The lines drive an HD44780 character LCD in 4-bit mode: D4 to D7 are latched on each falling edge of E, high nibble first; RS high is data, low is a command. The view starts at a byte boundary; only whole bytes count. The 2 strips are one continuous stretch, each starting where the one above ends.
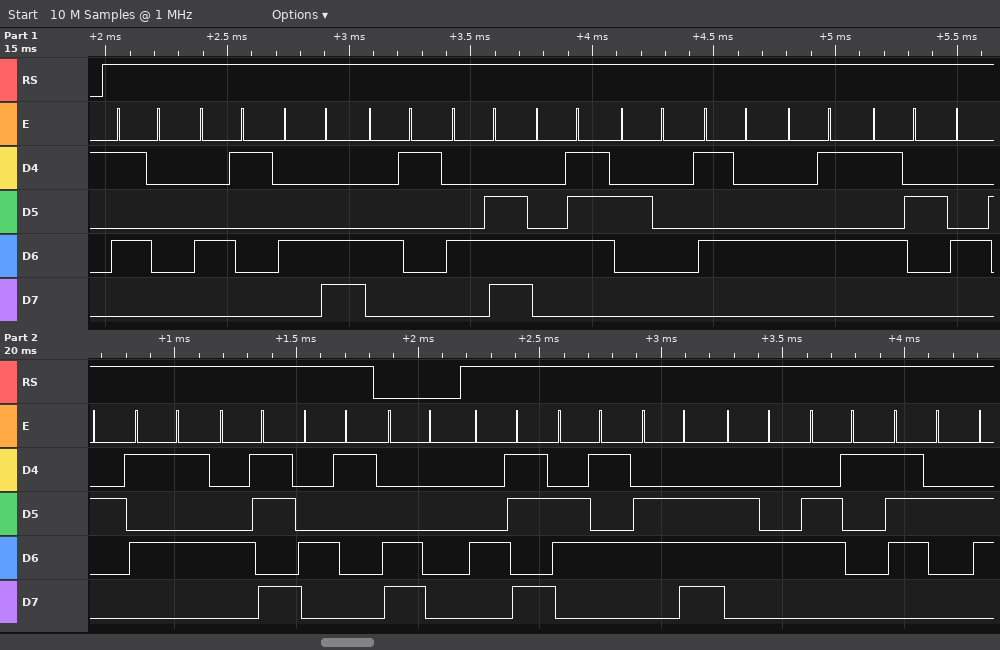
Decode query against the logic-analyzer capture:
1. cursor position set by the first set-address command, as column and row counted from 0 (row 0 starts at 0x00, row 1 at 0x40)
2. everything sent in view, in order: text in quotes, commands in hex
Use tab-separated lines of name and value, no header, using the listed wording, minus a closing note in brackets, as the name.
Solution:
cursor position set by the first set-address command, as column and row counted from 0	column 0, row 1
everything sent in view, in order: text in quotes, commands in hex	"PALANG TERBUKA" 0xC0 "Kendar"
